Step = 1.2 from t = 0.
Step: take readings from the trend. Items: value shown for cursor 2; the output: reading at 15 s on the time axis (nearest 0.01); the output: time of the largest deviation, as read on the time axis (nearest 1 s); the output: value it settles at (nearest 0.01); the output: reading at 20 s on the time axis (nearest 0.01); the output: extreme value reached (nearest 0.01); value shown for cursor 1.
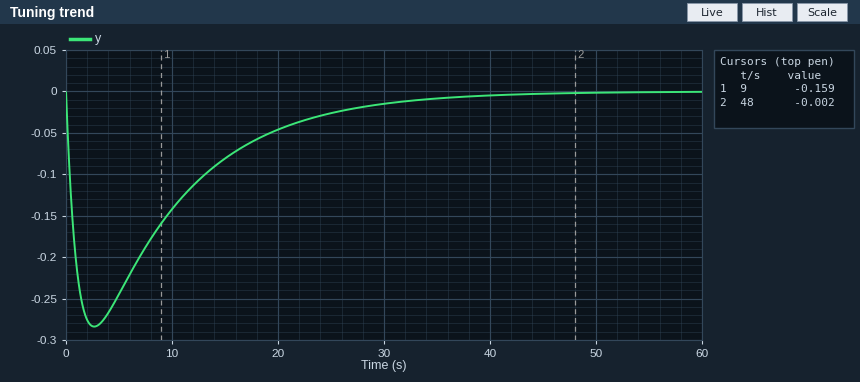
-0.002
-0.08
3 s
0.00
-0.05
-0.28
-0.159
